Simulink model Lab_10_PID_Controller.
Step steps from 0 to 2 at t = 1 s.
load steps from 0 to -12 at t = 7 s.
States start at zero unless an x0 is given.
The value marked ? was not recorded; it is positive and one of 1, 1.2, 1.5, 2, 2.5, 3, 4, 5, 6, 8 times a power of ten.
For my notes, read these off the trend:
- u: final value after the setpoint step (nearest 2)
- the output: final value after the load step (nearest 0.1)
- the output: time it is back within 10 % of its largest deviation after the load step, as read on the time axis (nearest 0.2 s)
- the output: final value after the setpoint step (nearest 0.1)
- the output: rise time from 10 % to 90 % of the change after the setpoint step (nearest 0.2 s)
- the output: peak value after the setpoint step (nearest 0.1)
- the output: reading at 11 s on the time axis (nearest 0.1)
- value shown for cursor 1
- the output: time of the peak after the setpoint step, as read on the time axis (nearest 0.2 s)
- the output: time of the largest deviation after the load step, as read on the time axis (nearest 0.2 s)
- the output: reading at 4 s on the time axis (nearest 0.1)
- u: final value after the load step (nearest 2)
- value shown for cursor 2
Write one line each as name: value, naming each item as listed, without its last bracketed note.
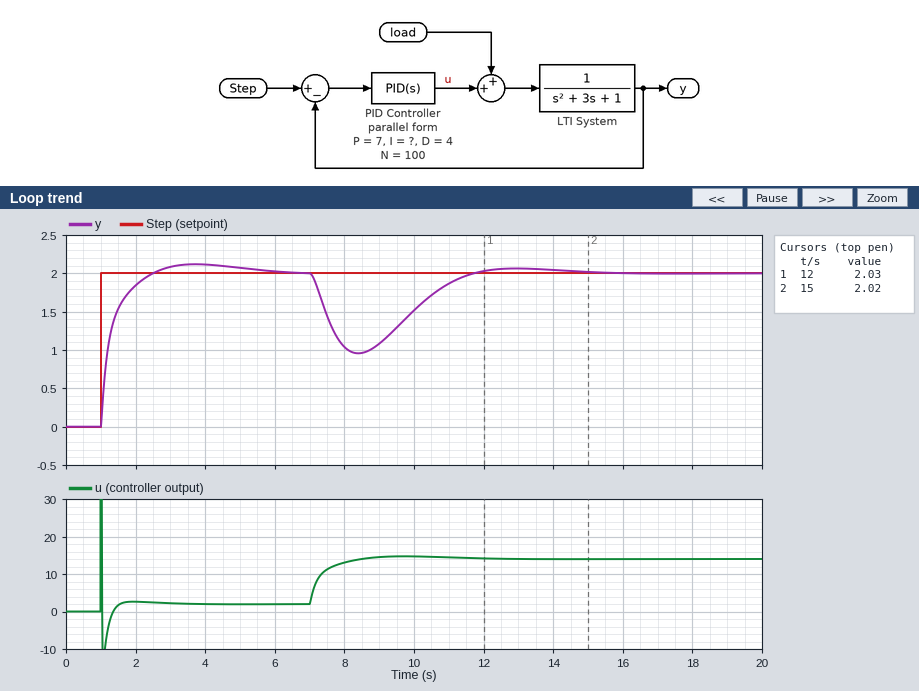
u: final value after the setpoint step: 2
the output: final value after the load step: 2.0
the output: time it is back within 10 % of its largest deviation after the load step, as read on the time axis: 11.2 s
the output: final value after the setpoint step: 2.0
the output: rise time from 10 % to 90 % of the change after the setpoint step: 0.8 s
the output: peak value after the setpoint step: 2.1
the output: reading at 11 s on the time axis: 1.9
value shown for cursor 1: 2.03
the output: time of the peak after the setpoint step, as read on the time axis: 3.8 s
the output: time of the largest deviation after the load step, as read on the time axis: 8.4 s
the output: reading at 4 s on the time axis: 2.1
u: final value after the load step: 14
value shown for cursor 2: 2.02
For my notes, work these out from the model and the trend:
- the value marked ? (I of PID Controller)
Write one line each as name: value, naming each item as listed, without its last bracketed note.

the value marked ?: 5
